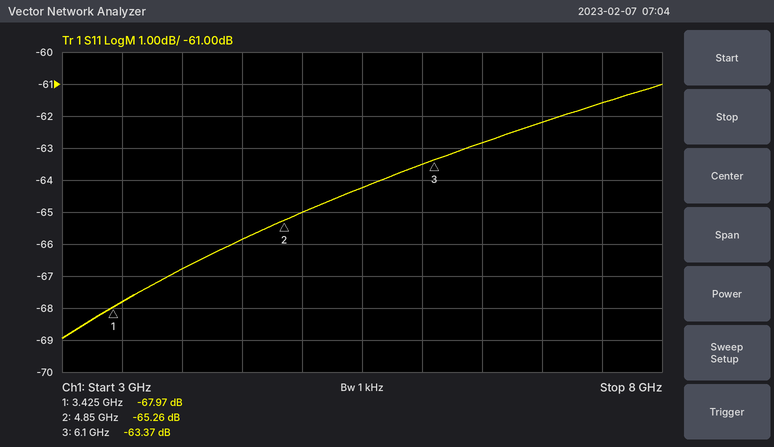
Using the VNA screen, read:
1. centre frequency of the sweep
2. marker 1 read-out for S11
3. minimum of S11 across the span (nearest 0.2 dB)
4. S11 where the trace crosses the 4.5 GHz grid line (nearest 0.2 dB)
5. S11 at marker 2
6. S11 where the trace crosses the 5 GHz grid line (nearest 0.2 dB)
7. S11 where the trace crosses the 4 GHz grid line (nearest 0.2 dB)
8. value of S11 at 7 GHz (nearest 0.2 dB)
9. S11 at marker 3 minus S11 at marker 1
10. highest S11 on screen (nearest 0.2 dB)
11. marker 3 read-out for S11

5.5 GHz
-67.97 dB
-69.0 dB
-65.8 dB
-65.26 dB
-65.0 dB
-66.8 dB
-62.2 dB
4.60 dB
-61.0 dB
-63.37 dB
